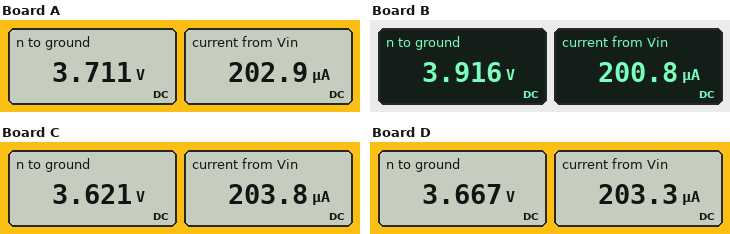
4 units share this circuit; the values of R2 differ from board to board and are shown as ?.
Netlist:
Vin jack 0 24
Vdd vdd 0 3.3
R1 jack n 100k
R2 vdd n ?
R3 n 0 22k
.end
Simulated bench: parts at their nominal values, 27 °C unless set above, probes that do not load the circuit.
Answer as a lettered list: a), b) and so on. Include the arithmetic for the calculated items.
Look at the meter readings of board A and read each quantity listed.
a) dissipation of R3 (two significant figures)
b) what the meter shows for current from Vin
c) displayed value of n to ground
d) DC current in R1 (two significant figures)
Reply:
a) (3.711 V)^2 / 22 kΩ = 630 µW
b) 202.9 µA
c) 3.711 V
d) (24 V - 3.711 V) / 100 kΩ = 200 µA
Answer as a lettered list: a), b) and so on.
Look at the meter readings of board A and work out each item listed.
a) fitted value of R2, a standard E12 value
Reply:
a) 12 kΩ
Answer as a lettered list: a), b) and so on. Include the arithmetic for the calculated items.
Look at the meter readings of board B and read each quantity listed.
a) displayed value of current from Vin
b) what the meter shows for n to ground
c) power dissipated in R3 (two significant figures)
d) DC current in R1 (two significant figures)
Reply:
a) 200.8 µA
b) 3.916 V
c) (3.916 V)^2 / 22 kΩ = 700 µW
d) (24 V - 3.916 V) / 100 kΩ = 200 µA
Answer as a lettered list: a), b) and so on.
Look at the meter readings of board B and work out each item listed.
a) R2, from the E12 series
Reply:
a) 27 kΩ
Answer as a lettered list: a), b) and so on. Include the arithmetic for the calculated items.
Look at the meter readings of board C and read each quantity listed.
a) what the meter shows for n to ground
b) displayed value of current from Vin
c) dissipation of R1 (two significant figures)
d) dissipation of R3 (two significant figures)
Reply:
a) 3.621 V
b) 203.8 µA
c) (24 V - 3.621 V)^2 / 100 kΩ = 4.2 mW
d) (3.621 V)^2 / 22 kΩ = 600 µW
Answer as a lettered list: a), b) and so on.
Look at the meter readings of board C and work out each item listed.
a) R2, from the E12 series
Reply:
a) 8.2 kΩ
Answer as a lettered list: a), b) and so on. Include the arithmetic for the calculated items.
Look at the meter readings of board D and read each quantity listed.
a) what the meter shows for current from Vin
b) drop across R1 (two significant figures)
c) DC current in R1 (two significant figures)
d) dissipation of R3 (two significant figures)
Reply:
a) 203.3 µA
b) 24 V - 3.667 V = 20 V
c) (24 V - 3.667 V) / 100 kΩ = 200 µA
d) (3.667 V)^2 / 22 kΩ = 610 µW
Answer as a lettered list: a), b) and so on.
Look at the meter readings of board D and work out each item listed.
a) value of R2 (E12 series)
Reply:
a) 10 kΩ
